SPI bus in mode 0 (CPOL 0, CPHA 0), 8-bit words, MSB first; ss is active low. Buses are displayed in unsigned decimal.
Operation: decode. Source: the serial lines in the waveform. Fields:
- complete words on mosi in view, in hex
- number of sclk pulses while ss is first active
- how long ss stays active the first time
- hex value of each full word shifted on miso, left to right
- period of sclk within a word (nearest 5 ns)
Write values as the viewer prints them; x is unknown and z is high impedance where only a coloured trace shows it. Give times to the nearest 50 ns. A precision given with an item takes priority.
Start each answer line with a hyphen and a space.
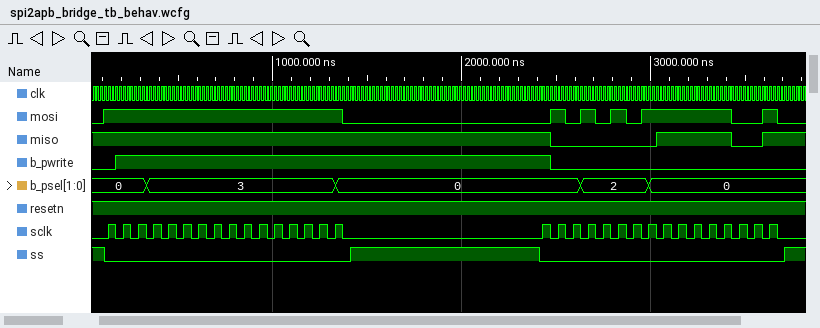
- FF, FF, 55, F9
- 16
- 1300 ns
- FF, FF, 80, F9
- 80 ns
